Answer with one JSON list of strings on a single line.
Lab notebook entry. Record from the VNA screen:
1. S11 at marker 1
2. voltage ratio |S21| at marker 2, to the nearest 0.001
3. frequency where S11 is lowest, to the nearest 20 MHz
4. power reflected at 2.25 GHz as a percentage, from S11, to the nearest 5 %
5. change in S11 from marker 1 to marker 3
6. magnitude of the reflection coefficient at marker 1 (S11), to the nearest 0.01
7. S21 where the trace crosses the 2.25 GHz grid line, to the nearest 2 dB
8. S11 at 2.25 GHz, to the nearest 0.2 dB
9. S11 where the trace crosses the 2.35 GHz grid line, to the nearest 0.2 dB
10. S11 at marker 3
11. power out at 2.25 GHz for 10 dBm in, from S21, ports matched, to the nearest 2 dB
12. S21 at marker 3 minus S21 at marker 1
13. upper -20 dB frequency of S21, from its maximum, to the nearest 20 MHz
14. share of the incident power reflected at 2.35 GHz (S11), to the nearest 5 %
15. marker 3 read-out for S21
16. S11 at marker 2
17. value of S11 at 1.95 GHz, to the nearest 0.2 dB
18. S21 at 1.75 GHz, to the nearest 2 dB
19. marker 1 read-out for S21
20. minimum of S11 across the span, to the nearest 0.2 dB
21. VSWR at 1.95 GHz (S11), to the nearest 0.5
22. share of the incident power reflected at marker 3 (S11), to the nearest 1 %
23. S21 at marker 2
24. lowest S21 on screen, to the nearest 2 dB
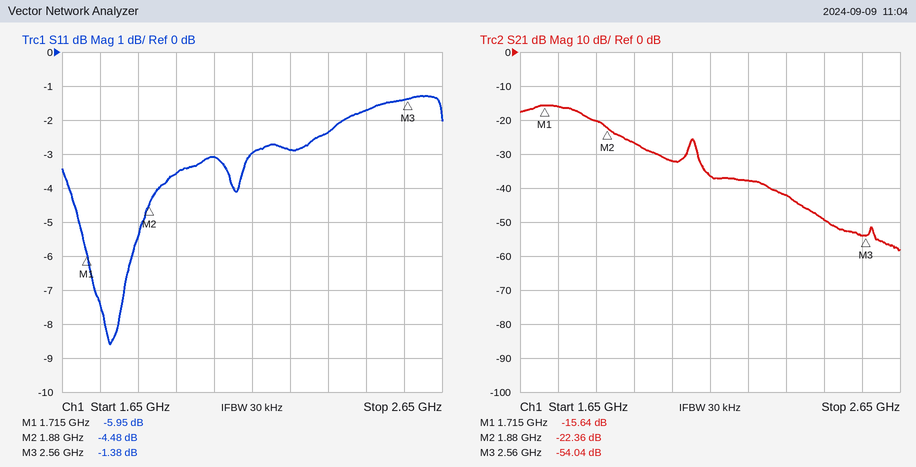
["-5.95 dB", "0.076", "1.78 GHz", "50 %", "4.57 dB", "0.50", "-38 dB", "-2.8 dB", "-2.4 dB", "-1.38 dB", "-28 dBm", "-38.40 dB", "2.14 GHz", "60 %", "-54.04 dB", "-4.48 dB", "-3.6 dB", "-16 dB", "-15.64 dB", "-8.6 dB", "5.0", "73 %", "-22.36 dB", "-58 dB"]
